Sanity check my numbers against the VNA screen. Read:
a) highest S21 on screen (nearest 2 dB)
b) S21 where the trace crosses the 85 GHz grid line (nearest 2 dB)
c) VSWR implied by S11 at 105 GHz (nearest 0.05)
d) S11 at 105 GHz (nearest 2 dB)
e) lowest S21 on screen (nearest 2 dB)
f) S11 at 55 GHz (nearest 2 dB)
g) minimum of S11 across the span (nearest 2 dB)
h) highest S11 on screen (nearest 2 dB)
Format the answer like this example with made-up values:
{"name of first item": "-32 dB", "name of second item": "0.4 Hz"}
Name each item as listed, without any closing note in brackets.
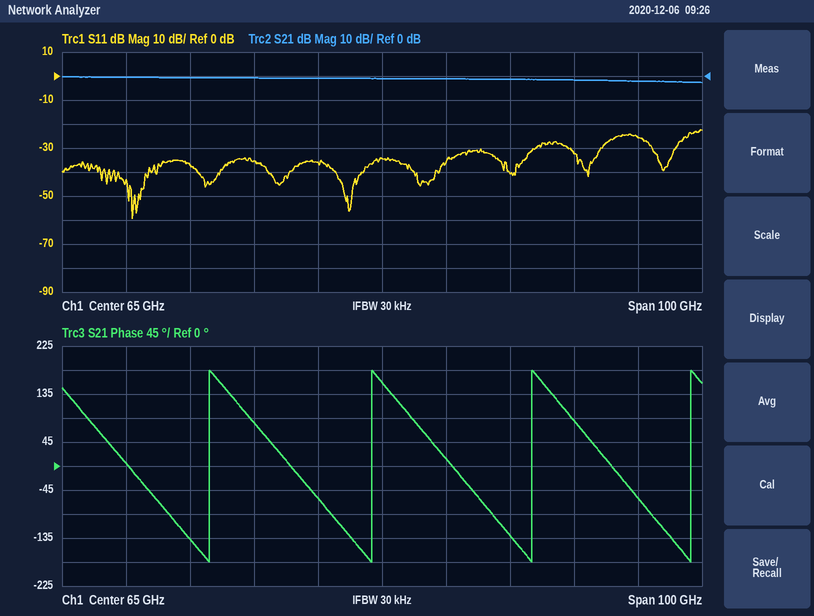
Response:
{"highest S21 on screen": "0 dB", "S21 where the trace crosses the 85 GHz grid line": "-2 dB", "VSWR implied by S11 at 105 GHz": "1.10", "S11 at 105 GHz": "-26 dB", "lowest S21 on screen": "-2 dB", "S11 at 55 GHz": "-36 dB", "minimum of S11 across the span": "-60 dB", "highest S11 on screen": "-22 dB"}
